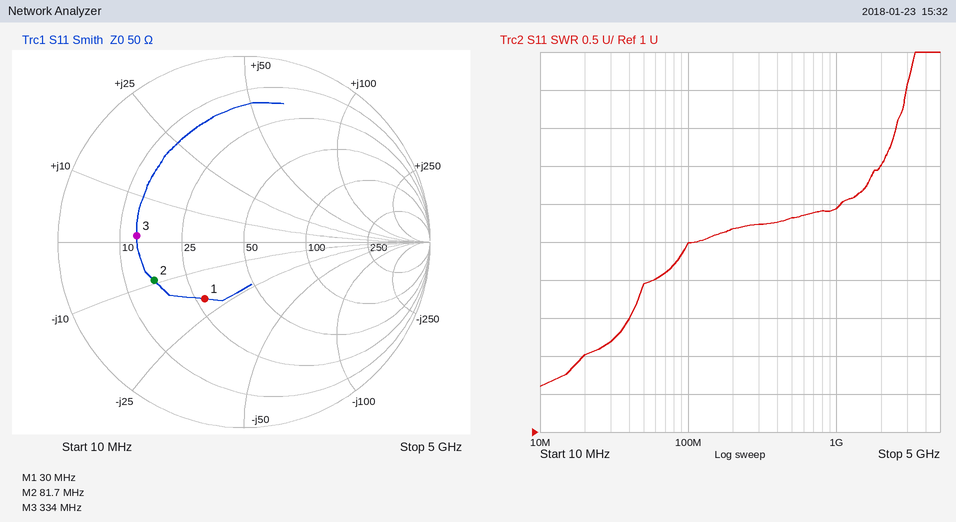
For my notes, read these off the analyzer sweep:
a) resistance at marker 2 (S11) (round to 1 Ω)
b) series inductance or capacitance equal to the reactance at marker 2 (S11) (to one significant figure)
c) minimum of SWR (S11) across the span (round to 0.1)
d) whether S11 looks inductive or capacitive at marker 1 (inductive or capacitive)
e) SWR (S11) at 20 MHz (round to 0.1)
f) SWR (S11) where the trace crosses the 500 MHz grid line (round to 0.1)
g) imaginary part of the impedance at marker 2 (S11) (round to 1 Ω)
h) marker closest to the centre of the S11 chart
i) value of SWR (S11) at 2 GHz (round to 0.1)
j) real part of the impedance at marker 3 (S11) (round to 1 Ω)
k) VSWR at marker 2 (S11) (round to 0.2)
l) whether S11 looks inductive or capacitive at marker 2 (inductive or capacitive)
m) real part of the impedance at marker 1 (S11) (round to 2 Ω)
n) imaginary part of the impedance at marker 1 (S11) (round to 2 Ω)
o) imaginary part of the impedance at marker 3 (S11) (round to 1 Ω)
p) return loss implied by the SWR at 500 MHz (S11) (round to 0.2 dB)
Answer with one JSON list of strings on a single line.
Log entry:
["16 Ω", "200 pF", "1.6", "capacitive", "2.0", "3.8", "-9 Ω", "marker 1", "4.5", "13 Ω", "3.2", "capacitive", "28 Ω", "-20 Ω", "+1 Ω", "4.6 dB"]
